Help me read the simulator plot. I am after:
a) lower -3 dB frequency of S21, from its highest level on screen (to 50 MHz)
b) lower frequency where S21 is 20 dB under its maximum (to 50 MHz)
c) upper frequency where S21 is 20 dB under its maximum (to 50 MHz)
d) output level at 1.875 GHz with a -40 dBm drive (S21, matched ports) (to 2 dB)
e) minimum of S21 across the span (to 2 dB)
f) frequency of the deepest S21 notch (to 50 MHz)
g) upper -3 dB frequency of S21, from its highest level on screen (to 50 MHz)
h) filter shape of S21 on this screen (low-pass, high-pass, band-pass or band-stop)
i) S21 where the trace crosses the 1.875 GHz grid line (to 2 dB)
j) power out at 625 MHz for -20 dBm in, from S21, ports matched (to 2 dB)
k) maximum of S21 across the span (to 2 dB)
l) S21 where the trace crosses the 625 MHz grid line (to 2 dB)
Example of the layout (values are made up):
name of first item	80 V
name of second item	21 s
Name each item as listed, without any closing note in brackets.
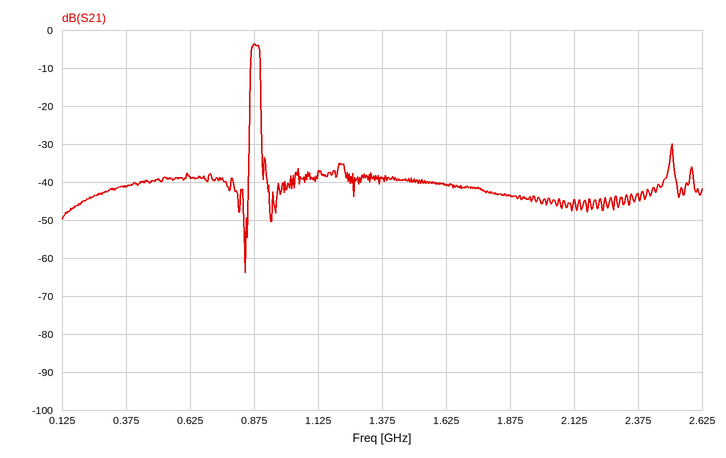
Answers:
lower -3 dB frequency of S21, from its highest level on screen	850 MHz
lower frequency where S21 is 20 dB under its maximum	850 MHz
upper frequency where S21 is 20 dB under its maximum	900 MHz
output level at 1.875 GHz with a -40 dBm drive (S21, matched ports)	-84 dBm
minimum of S21 across the span	-64 dB
frequency of the deepest S21 notch	850 MHz
upper -3 dB frequency of S21, from its highest level on screen	900 MHz
filter shape of S21 on this screen	band-pass
S21 where the trace crosses the 1.875 GHz grid line	-44 dB
power out at 625 MHz for -20 dBm in, from S21, ports matched	-58 dBm
maximum of S21 across the span	-4 dB
S21 where the trace crosses the 625 MHz grid line	-38 dB
